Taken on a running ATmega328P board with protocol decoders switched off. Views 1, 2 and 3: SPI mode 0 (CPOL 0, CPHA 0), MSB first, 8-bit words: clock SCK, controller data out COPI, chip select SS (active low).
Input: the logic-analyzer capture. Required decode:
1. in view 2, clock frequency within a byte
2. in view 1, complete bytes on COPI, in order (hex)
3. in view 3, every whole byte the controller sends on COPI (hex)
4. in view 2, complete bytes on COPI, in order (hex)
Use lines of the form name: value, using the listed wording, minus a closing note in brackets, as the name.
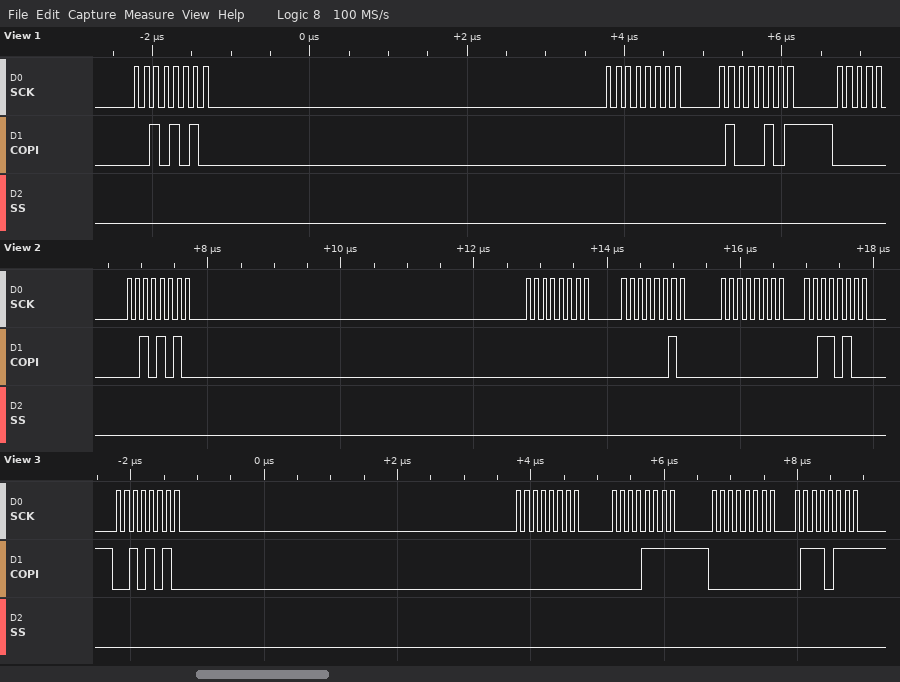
in view 2, clock frequency within a byte: 8 MHz
in view 1, complete bytes on COPI, in order: 2A 00 45
in view 3, every whole byte the controller sends on COPI: 0x2A 0x00 0x0F 0x00 0x77
in view 2, complete bytes on COPI, in order: 2A 00 02 00 34
